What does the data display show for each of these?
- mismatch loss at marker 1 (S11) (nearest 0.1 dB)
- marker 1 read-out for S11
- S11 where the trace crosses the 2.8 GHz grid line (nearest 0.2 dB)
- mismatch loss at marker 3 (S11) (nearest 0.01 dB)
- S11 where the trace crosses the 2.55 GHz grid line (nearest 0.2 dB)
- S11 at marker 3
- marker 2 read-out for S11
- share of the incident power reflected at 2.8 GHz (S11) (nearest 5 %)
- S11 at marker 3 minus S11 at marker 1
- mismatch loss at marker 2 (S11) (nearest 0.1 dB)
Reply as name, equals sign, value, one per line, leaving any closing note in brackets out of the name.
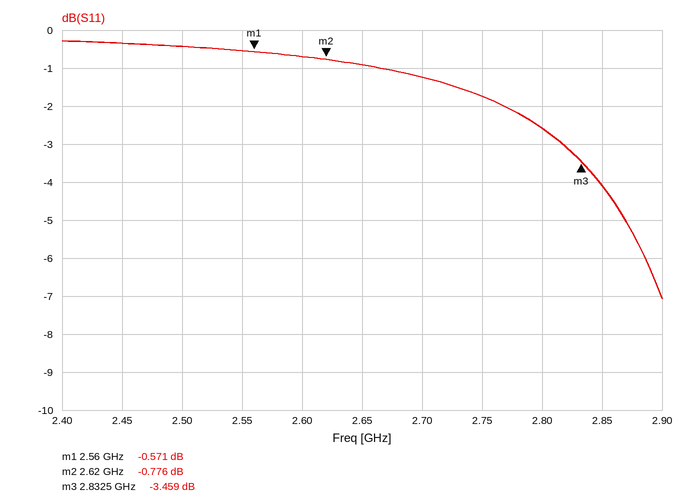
mismatch loss at marker 1 (S11) = 9.1 dB
marker 1 read-out for S11 = -0.571 dB
S11 where the trace crosses the 2.8 GHz grid line = -2.6 dB
mismatch loss at marker 3 (S11) = 2.60 dB
S11 where the trace crosses the 2.55 GHz grid line = -0.6 dB
S11 at marker 3 = -3.459 dB
marker 2 read-out for S11 = -0.776 dB
share of the incident power reflected at 2.8 GHz (S11) = 55 %
S11 at marker 3 minus S11 at marker 1 = -2.888 dB
mismatch loss at marker 2 (S11) = 7.9 dB
